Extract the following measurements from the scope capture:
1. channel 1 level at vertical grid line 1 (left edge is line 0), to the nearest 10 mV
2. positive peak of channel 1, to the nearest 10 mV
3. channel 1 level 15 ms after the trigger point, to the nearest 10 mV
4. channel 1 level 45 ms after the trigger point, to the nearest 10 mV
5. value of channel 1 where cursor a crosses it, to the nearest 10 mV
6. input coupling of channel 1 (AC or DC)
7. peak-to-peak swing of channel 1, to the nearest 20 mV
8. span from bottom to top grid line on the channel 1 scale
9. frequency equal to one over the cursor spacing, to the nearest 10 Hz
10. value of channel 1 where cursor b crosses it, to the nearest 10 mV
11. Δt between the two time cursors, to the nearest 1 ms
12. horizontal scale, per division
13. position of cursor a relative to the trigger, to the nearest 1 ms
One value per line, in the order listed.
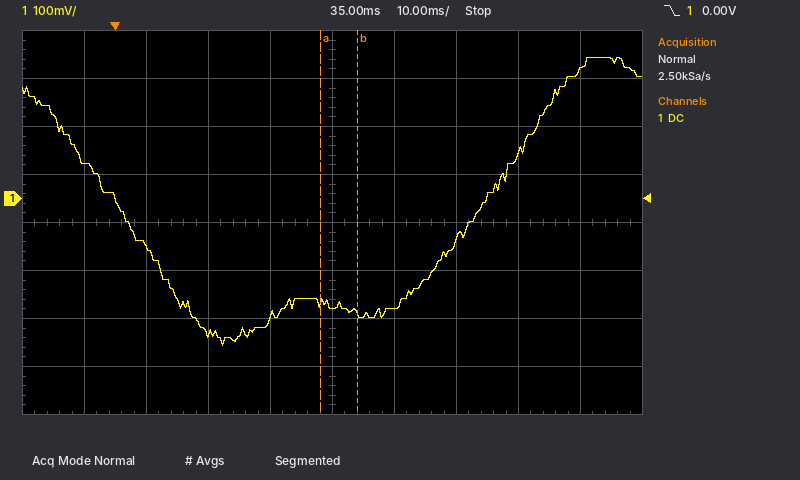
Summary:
70 mV
290 mV
-280 mV
-230 mV
-220 mV
DC
600 mV
800 mV
170 Hz
-240 mV
6 ms
10 ms
+33 ms
